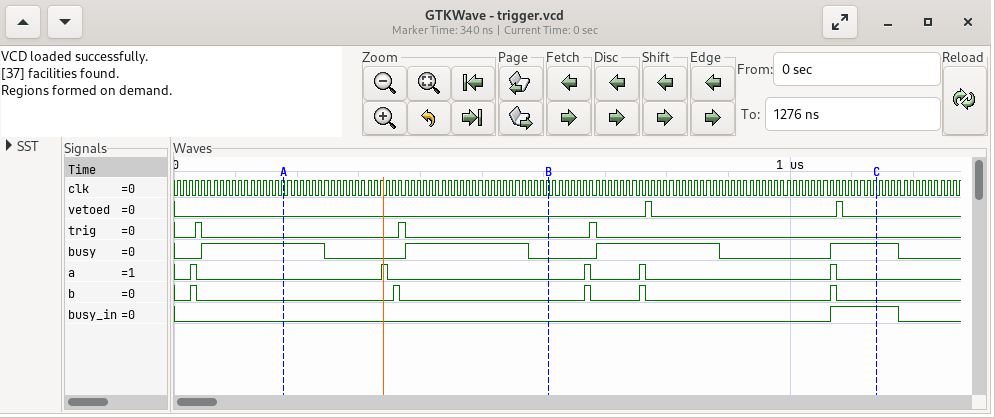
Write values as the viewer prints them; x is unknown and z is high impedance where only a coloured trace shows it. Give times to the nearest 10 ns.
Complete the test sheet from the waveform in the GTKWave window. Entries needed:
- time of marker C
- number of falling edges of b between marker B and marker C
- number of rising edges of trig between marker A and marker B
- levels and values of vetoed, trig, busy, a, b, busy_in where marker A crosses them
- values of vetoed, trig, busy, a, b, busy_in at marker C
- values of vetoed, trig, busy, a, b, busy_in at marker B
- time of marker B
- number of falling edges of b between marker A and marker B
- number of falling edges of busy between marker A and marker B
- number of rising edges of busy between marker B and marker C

1140 ns
3
1
vetoed=0, trig=0, busy=1, a=0, b=0, busy_in=0
vetoed=0, trig=0, busy=1, a=0, b=0, busy_in=1
vetoed=0, trig=0, busy=0, a=0, b=0, busy_in=0
610 ns
1
2
2
